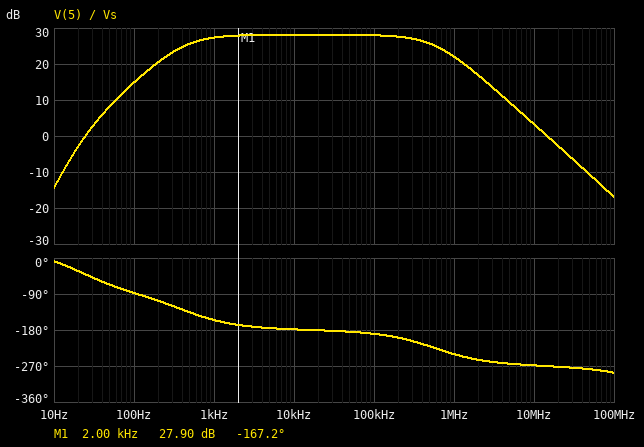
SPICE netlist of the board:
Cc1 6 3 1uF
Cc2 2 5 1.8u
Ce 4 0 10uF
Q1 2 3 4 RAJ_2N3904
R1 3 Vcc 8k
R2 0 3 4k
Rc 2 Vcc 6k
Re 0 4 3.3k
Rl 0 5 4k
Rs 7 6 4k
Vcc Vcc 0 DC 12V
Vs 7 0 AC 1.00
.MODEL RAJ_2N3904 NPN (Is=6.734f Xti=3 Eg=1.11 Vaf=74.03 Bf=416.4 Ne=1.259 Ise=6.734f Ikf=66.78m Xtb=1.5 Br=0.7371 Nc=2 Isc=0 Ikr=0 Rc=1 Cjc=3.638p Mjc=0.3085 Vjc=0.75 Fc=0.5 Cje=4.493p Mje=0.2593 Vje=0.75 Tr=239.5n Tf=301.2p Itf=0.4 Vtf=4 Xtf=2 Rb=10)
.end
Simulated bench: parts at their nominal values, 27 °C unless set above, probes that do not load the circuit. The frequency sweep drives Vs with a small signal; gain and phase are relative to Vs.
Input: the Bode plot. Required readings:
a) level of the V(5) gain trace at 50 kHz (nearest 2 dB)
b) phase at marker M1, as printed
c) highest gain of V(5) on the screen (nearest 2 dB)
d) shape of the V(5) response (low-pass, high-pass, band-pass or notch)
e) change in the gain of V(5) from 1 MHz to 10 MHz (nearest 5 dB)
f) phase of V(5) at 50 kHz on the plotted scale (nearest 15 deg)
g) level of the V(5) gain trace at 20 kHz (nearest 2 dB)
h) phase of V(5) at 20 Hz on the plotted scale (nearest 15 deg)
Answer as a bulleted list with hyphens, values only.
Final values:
- 28 dB
- -167.2 deg
- 28 dB
- band-pass
- -20 dB
- -180 deg
- 28 dB
- -30 deg
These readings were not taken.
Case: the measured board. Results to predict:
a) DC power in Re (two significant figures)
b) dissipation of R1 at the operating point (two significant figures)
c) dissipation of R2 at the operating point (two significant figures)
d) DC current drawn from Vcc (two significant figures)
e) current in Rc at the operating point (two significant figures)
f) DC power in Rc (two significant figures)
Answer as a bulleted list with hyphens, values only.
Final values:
- 3.3 mW
- 8.0 mW
- 4.0 mW
- 2.0 mA
- 1.0 mA
- 6.0 mW
